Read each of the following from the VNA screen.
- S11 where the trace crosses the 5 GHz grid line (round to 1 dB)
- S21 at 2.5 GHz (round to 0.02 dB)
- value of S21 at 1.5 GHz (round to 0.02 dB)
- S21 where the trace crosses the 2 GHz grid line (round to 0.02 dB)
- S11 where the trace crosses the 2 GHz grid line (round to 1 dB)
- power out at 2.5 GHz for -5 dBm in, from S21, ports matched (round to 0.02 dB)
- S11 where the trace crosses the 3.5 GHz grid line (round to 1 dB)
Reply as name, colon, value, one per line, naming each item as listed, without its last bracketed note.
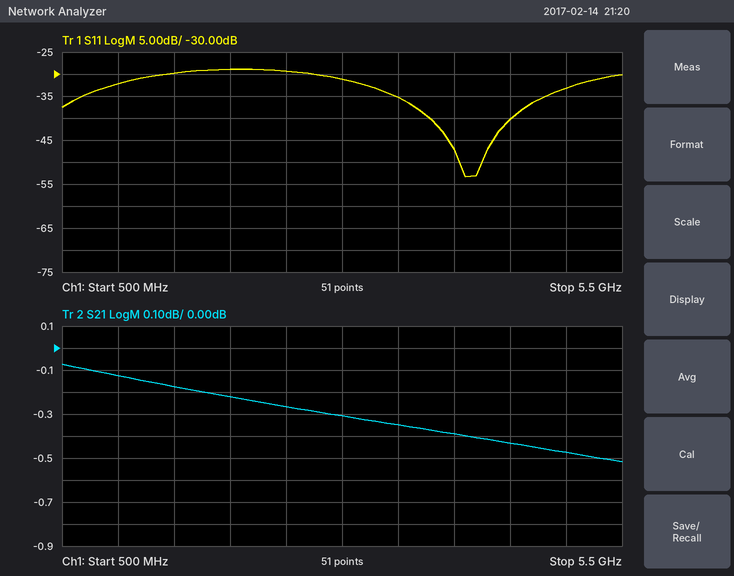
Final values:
S11 where the trace crosses the 5 GHz grid line: -33 dB
S21 at 2.5 GHz: -0.26 dB
value of S21 at 1.5 GHz: -0.18 dB
S21 where the trace crosses the 2 GHz grid line: -0.22 dB
S11 where the trace crosses the 2 GHz grid line: -29 dB
power out at 2.5 GHz for -5 dBm in, from S21, ports matched: -5.26 dBm
S11 where the trace crosses the 3.5 GHz grid line: -35 dB
